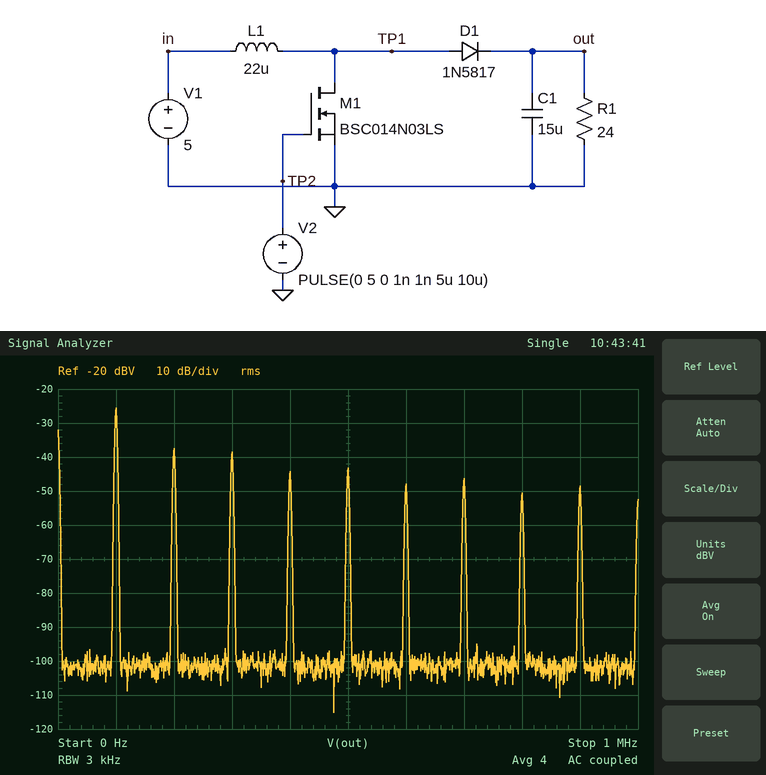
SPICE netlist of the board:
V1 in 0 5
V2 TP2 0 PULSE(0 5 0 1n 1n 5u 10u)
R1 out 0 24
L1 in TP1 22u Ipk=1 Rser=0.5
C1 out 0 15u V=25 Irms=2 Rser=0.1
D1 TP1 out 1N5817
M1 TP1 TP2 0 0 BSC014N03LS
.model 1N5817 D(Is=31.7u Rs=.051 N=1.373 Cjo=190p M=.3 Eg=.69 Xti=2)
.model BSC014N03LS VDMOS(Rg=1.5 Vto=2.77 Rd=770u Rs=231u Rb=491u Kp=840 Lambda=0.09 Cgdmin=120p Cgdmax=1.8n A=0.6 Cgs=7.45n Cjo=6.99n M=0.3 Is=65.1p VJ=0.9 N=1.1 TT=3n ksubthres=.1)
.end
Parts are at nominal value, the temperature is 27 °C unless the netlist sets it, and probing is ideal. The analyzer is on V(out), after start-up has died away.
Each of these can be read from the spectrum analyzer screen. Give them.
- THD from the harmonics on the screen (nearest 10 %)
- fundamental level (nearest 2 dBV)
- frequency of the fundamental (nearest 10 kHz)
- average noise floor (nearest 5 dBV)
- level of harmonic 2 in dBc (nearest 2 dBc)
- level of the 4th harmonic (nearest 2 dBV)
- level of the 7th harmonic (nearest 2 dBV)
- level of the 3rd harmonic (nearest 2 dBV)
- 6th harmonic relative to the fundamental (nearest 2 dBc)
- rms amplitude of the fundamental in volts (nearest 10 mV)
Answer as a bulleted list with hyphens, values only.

- 40 %
- -26 dBV
- 100 kHz
- -100 dBV
- -12 dBc
- -44 dBV
- -46 dBV
- -38 dBV
- -22 dBc
- 50 mV
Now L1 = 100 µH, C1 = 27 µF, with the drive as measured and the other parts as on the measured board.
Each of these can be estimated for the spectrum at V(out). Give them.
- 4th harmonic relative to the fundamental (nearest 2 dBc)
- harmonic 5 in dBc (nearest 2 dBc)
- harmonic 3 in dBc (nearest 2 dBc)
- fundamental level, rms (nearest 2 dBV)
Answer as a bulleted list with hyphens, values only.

- -28 dBc
- -16 dBc
- -10 dBc
- -28 dBV
